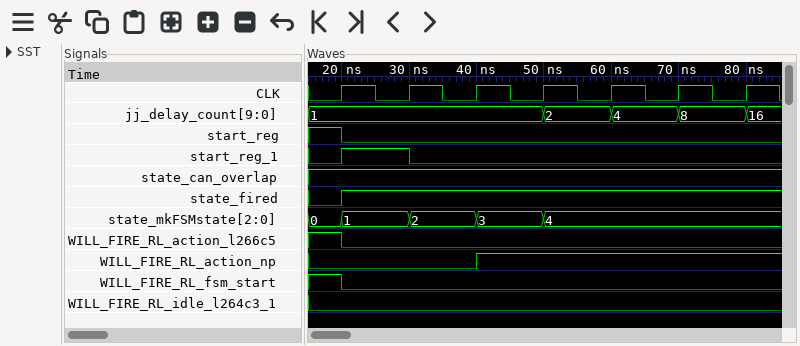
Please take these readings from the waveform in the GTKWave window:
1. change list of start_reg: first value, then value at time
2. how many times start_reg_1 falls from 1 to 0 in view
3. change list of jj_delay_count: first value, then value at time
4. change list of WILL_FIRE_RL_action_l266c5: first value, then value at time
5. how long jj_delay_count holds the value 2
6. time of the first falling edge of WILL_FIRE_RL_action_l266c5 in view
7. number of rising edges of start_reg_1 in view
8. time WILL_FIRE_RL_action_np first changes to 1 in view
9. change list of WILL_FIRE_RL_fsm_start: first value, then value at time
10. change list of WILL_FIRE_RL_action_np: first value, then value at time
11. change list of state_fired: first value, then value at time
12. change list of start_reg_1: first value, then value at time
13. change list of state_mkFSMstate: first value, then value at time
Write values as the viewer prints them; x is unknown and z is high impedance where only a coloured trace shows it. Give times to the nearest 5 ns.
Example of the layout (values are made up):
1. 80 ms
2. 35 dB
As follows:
1. 1, 0 at 20 ns
2. 1
3. 1, 2 at 50 ns, 4 at 60 ns, 8 at 70 ns, 16 at 80 ns
4. 1, 0 at 20 ns
5. 10 ns
6. 20 ns
7. 1
8. 40 ns
9. 1, 0 at 20 ns
10. 0, 1 at 40 ns
11. 0, 1 at 20 ns
12. 0, 1 at 20 ns, 0 at 30 ns
13. 0, 1 at 20 ns, 2 at 30 ns, 3 at 40 ns, 4 at 50 ns
